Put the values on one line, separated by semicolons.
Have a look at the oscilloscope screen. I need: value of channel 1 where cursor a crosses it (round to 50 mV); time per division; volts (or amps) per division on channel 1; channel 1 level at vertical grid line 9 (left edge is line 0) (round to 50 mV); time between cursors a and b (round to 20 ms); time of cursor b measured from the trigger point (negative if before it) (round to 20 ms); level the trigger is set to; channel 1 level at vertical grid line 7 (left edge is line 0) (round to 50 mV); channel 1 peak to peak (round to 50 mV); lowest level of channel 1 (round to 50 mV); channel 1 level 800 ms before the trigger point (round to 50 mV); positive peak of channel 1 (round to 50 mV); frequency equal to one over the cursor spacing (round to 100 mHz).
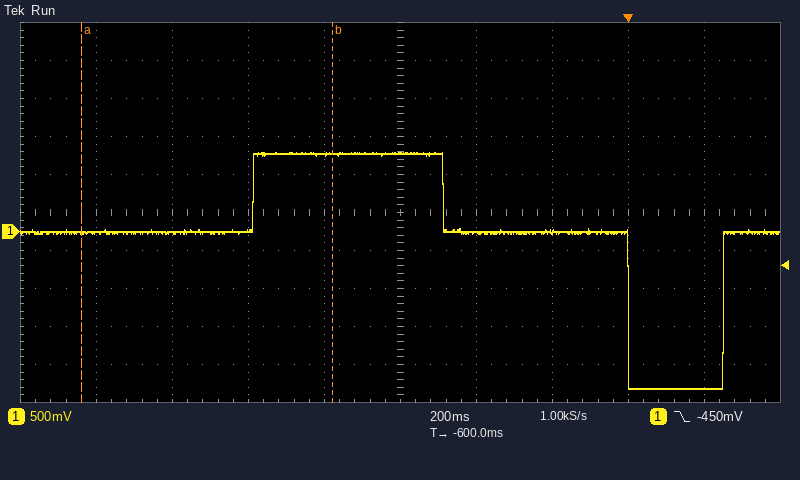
0 mV; 200 ms; 500 mV; -2.05 V; 660 ms; -780 ms; -450 mV; 0 mV; 3.10 V; -2.05 V; 1.00 V; 1.05 V; 1.5 Hz
